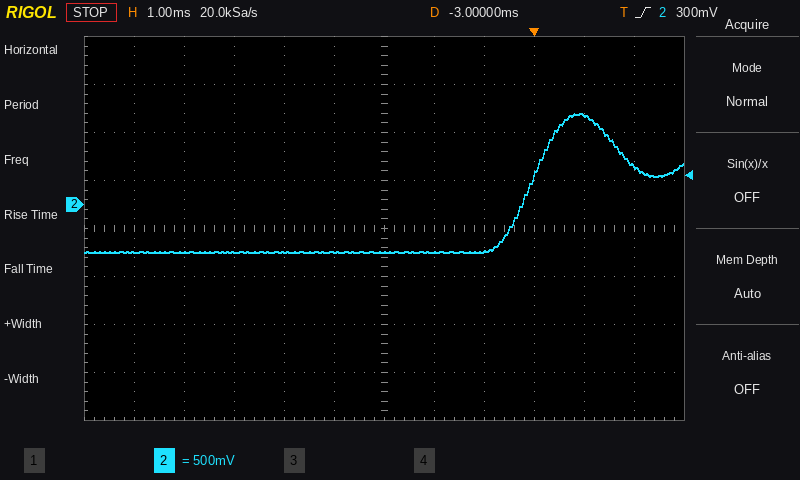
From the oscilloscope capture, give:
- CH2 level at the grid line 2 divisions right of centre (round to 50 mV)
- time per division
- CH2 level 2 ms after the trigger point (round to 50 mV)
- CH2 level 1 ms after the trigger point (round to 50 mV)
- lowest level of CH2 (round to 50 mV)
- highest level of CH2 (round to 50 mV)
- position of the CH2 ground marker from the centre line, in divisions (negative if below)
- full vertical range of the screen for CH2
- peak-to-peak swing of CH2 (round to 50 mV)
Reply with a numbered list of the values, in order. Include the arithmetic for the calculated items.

1. -500 mV
2. 1 ms
3. 400 mV
4. 950 mV
5. -500 mV
6. 950 mV
7. +0.5 div
8. 4 V
9. 950 mV − (-500 mV) = 1.45 V
